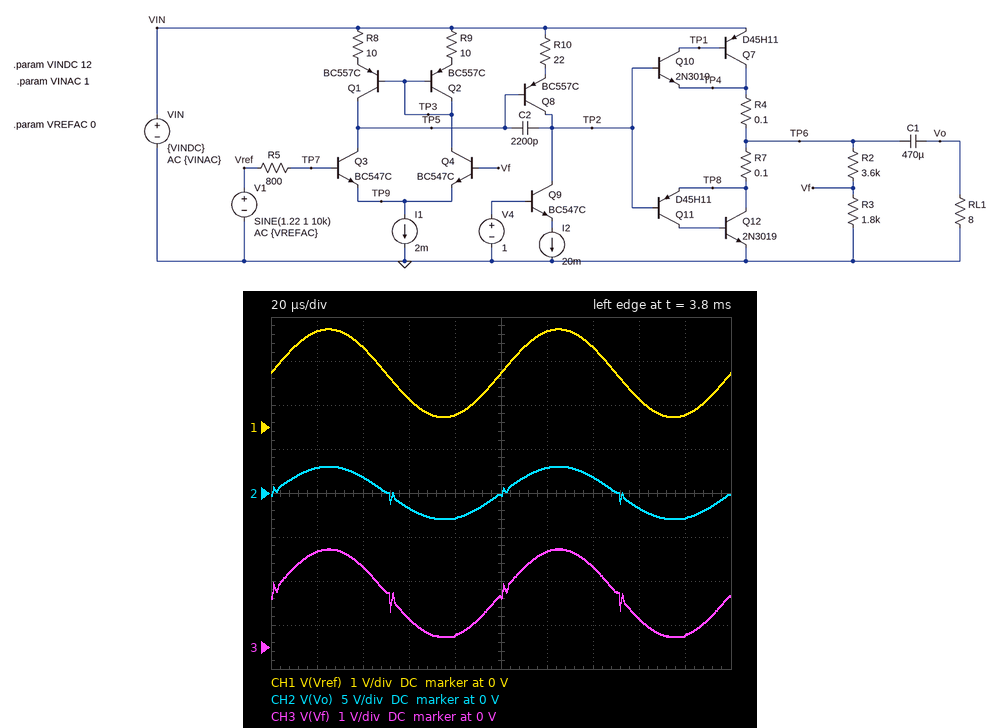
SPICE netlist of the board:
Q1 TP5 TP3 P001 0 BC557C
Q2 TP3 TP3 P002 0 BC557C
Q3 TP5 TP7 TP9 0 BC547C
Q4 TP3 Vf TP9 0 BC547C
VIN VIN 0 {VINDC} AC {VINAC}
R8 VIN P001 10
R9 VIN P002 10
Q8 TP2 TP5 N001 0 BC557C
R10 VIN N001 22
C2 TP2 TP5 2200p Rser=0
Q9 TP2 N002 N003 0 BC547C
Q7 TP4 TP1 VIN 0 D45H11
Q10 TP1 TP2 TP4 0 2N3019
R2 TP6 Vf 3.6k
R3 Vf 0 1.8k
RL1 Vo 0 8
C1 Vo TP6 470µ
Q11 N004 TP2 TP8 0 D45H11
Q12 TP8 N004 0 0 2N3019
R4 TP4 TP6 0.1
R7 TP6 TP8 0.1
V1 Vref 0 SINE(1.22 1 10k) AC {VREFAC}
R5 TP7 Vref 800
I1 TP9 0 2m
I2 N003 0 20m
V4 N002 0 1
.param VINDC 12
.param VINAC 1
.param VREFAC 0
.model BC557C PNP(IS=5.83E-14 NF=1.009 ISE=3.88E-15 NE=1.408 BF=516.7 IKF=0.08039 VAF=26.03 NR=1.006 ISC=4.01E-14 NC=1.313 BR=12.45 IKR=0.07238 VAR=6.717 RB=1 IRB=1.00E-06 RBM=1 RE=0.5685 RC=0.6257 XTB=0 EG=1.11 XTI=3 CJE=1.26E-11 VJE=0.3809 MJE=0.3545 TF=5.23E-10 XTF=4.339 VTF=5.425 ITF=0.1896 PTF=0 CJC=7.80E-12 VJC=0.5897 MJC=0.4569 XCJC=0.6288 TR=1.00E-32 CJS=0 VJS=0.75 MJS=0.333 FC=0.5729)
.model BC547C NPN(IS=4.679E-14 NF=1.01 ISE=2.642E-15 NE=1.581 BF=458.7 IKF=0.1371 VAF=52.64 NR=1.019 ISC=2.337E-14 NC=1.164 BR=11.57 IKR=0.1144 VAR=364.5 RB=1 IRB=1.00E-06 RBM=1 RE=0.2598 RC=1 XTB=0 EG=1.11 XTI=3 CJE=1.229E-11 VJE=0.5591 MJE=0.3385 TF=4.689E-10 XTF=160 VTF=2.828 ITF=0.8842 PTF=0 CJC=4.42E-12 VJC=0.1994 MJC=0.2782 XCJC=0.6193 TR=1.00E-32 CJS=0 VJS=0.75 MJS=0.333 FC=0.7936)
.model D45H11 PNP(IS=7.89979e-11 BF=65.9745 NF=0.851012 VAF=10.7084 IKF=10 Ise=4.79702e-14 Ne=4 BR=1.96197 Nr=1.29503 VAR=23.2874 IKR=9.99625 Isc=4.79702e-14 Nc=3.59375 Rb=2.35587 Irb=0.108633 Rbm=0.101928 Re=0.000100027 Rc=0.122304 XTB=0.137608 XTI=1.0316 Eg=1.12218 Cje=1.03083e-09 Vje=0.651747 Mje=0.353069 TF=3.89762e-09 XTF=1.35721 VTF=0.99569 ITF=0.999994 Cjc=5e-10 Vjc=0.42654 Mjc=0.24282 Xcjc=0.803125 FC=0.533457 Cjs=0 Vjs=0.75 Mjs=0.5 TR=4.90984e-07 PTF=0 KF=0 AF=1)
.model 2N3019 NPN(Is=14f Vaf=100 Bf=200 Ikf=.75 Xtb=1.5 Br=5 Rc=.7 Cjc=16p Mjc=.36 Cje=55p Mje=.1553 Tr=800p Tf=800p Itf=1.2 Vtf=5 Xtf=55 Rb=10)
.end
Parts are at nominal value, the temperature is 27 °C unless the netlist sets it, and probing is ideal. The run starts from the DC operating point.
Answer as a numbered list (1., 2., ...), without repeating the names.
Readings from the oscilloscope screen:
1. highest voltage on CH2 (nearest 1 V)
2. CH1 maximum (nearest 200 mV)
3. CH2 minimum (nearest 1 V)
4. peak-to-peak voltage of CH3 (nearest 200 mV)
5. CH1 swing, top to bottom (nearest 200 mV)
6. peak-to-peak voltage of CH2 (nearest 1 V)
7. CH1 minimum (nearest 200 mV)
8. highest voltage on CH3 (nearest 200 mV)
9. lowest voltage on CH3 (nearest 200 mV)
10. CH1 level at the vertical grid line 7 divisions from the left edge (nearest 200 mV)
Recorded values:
1. 3 V
2. 2.2 V
3. -3 V
4. 2.0 V
5. 2.0 V
6. 6 V
7. 200 mV
8. 2.2 V
9. 200 mV
10. 1.8 V
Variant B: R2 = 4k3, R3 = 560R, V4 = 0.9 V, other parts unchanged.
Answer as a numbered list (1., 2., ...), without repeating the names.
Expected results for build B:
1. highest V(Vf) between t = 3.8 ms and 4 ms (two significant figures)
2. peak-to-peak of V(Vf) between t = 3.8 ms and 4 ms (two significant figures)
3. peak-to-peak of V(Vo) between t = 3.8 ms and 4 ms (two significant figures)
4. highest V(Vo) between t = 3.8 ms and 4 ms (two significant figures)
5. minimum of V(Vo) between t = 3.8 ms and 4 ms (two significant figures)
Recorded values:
1. 1.2 V
2. 1.0 V
3. 8.9 V
4. 1.9 V
5. -7.0 V
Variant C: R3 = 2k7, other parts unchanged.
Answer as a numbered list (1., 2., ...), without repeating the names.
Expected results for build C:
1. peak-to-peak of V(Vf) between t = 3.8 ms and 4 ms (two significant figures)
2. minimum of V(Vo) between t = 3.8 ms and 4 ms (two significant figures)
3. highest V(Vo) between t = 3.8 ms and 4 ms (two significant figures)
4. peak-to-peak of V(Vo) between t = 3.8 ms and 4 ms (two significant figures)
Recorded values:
1. 1.9 V
2. -2.2 V
3. 2.3 V
4. 4.5 V
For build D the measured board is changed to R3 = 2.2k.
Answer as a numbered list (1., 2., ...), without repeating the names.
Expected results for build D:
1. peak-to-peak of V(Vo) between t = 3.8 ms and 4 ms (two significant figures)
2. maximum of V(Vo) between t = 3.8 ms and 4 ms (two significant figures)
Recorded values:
1. 5.2 V
2. 2.6 V
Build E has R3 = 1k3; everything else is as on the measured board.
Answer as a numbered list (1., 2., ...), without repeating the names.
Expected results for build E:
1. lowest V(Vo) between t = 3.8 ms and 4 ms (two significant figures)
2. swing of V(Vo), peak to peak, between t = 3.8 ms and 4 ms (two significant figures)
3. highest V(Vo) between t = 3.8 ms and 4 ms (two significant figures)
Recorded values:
1. -3.8 V
2. 7.5 V
3. 3.8 V
